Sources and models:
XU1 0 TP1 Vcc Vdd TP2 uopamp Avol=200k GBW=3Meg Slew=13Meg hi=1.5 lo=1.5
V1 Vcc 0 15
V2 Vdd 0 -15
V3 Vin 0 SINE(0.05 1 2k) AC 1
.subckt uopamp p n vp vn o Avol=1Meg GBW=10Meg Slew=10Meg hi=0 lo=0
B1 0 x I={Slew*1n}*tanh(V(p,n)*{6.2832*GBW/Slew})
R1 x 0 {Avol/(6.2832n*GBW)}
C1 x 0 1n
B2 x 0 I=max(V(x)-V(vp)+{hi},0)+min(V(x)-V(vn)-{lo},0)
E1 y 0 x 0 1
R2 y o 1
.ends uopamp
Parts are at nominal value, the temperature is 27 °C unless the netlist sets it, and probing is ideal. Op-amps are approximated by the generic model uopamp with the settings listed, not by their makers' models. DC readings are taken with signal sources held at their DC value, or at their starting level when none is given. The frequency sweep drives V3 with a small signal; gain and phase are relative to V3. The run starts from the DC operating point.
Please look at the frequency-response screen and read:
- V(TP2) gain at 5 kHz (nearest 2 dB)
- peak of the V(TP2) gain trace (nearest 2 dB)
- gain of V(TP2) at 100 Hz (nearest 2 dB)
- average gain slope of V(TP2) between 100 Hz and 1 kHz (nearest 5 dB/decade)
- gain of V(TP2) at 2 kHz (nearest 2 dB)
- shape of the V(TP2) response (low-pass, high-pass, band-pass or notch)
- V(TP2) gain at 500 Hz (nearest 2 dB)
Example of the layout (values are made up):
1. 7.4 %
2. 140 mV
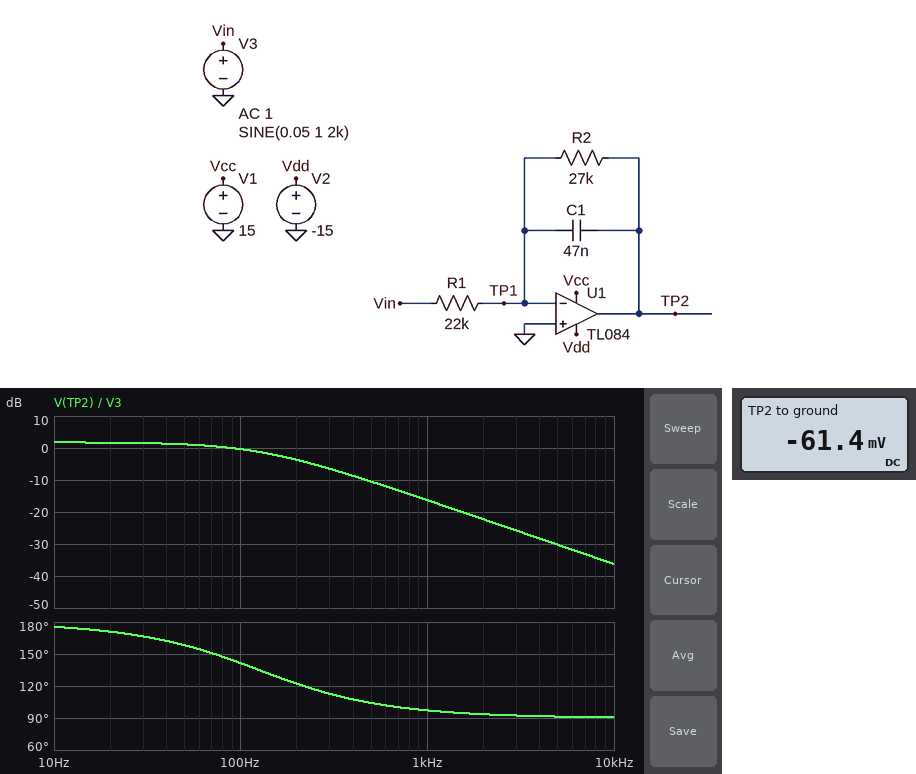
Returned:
1. -30 dB
2. 2 dB
3. 0 dB
4. -15 dB/decade
5. -22 dB
6. low-pass
7. -10 dB
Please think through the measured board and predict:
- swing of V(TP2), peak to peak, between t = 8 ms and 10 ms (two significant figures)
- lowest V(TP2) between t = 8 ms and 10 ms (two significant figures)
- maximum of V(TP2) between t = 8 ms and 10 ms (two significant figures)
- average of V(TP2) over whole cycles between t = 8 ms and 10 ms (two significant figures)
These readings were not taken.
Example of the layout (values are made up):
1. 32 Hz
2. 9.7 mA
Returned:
1. 150 mV
2. -140 mV
3. 15 mV
4. -61 mV
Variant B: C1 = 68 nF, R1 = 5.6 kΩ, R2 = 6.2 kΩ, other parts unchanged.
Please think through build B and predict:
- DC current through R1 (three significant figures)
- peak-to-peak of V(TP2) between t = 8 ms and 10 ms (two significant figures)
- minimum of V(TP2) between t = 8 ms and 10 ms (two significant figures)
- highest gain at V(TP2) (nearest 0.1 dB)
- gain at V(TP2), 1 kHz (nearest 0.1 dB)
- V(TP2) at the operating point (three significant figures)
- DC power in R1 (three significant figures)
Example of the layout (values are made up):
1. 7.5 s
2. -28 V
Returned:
1. 8.93 µA
2. 410 mV
3. -260 mV
4. 0.9 dB
5. -8.2 dB
6. -55.4 mV
7. 446 nW
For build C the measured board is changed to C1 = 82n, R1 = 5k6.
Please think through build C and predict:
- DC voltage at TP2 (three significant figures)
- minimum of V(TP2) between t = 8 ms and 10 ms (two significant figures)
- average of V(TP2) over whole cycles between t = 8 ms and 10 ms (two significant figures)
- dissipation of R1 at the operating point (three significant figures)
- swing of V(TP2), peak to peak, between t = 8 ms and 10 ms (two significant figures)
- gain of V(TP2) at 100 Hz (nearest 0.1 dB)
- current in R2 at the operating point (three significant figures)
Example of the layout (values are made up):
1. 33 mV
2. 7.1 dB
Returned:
1. -241 mV
2. -420 mV
3. -240 mV
4. 446 nW
5. 350 mV
6. 9.0 dB
7. 8.93 µA
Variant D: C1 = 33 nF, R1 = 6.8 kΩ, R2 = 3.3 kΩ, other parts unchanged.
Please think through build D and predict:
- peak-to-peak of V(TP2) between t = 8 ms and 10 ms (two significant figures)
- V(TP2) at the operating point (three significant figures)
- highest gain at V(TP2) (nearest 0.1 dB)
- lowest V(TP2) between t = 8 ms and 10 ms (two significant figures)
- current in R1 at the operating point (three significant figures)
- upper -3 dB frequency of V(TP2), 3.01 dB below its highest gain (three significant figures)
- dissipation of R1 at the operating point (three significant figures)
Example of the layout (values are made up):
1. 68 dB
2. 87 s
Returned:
1. 570 mV
2. -24.3 mV
3. -6.3 dB
4. -310 mV
5. 7.35 µA
6. 1.46 kHz
7. 368 nW
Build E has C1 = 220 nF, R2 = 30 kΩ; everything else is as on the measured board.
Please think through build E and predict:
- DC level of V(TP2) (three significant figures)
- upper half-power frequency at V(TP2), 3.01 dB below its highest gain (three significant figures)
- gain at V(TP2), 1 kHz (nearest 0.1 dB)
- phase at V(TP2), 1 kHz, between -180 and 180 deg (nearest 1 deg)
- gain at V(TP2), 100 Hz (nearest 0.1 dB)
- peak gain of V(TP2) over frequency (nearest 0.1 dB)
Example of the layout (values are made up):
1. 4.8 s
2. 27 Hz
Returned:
1. -68.2 mV
2. 24.1 Hz
3. -29.7 dB
4. 91 deg
5. -9.9 dB
6. 2.7 dB
